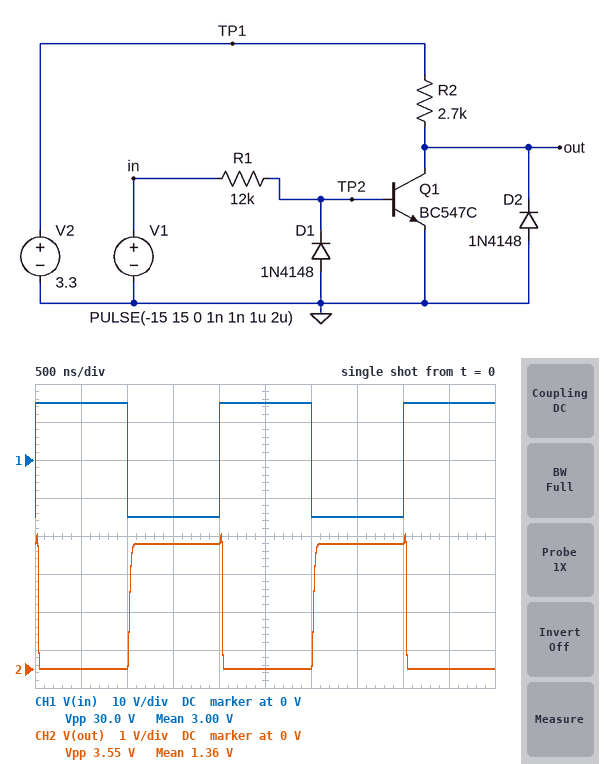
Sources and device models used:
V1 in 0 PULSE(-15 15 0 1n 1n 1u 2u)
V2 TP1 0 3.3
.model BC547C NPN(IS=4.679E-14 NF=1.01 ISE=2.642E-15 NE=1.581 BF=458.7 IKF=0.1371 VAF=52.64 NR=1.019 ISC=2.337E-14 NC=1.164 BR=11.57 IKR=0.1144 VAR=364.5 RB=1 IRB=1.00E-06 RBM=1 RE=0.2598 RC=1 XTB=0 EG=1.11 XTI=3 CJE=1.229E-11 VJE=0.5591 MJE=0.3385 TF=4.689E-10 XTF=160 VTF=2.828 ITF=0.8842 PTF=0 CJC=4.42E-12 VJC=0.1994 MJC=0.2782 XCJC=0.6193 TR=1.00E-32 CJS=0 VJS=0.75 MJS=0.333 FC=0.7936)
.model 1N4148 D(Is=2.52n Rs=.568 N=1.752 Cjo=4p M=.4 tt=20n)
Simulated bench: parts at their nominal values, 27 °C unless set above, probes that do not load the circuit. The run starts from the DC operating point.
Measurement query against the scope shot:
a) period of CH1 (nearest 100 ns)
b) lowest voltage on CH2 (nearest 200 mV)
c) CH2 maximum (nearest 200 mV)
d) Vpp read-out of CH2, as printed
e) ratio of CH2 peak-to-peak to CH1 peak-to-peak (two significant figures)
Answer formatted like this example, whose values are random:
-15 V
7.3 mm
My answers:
2.0 µs
0 V
3.6 V
3.55 V
0.12
